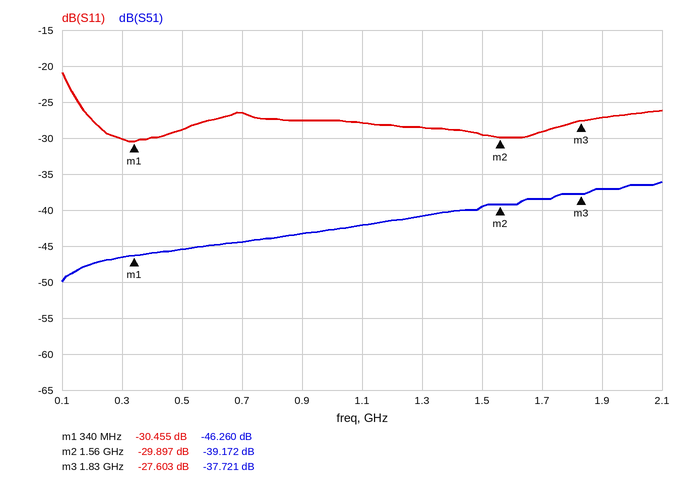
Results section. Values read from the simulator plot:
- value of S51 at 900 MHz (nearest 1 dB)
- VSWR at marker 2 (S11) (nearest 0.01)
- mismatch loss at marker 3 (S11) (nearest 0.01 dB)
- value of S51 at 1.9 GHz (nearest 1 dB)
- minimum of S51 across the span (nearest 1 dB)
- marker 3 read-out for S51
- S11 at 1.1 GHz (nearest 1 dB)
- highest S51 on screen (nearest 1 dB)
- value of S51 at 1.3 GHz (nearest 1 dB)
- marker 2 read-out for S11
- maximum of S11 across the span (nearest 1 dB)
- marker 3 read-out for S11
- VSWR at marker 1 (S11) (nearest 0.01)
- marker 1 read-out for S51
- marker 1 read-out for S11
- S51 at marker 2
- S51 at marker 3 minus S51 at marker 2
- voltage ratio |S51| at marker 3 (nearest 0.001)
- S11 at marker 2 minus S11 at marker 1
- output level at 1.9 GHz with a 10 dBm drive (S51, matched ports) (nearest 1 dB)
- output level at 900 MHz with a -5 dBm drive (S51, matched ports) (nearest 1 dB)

-43 dB
1.07
0.01 dB
-37 dB
-50 dB
-37.721 dB
-28 dB
-36 dB
-41 dB
-29.897 dB
-21 dB
-27.603 dB
1.06
-46.260 dB
-30.455 dB
-39.172 dB
1.451 dB
0.013
0.558 dB
-27 dBm
-48 dBm
